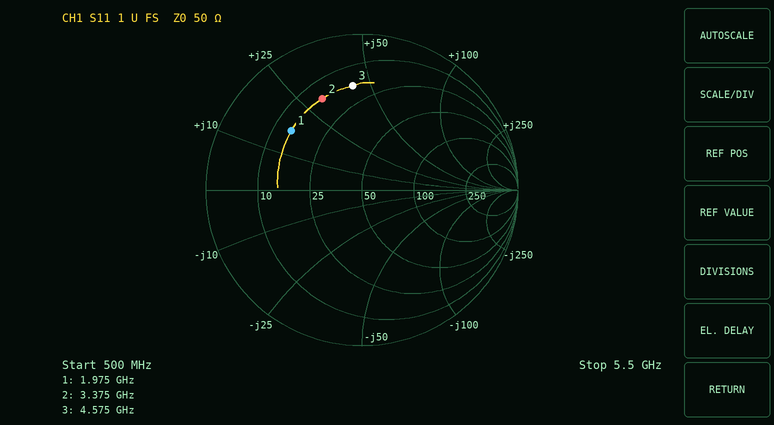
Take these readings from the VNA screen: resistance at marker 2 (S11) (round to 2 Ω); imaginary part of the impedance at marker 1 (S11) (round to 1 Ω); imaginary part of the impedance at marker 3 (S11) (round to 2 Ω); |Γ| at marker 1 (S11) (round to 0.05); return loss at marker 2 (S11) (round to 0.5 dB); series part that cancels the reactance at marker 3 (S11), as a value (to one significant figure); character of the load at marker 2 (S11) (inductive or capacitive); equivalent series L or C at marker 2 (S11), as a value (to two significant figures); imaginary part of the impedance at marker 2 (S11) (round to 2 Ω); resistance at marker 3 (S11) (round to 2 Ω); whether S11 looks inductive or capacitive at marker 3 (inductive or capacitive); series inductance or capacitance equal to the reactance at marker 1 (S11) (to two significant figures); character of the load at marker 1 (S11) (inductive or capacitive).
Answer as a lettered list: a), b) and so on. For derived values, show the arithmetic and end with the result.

a) 16 Ω
b) +17 Ω
c) +42 Ω
d) 0.60
e) 4.0 dB
f) C = 1/(2π × 4.575 GHz × 42 Ω) ≈ 828 fF, so 800 fF to one significant figure
g) inductive
h) L = 30 Ω/(2π × 3.375 GHz) ≈ 1.4 nH
i) +30 Ω
j) 18 Ω
k) inductive
l) L = 17 Ω/(2π × 1.975 GHz) ≈ 1.4 nH
m) inductive
